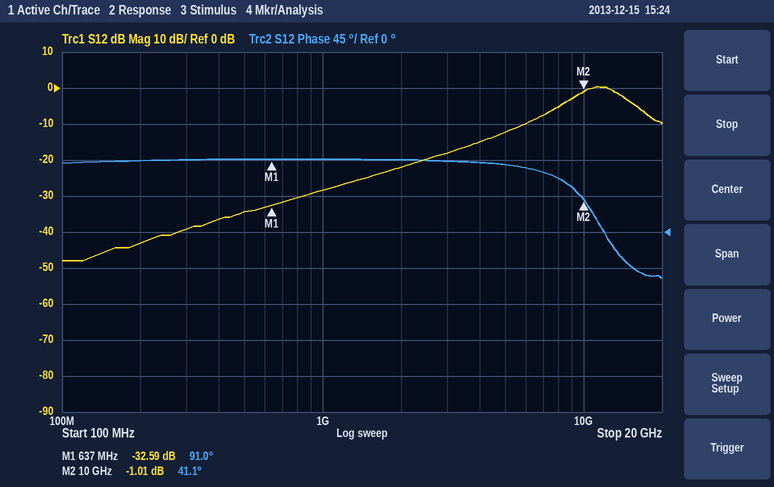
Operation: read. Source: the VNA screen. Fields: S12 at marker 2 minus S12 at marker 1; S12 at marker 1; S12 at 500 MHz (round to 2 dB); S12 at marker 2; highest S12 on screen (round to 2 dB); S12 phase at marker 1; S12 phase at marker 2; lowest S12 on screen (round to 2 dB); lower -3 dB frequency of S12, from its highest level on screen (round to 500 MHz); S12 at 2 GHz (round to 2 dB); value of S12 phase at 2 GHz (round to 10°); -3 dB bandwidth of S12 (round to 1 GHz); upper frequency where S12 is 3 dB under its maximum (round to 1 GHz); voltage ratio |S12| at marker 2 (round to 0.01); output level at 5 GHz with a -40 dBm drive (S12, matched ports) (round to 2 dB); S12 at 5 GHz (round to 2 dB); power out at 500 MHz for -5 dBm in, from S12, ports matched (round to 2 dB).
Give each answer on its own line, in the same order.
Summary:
31.58 dB
-32.59 dB
-34 dB
-1.01 dB
0 dB
91.0°
41.1°
-48 dB
9.0 GHz
-22 dB
90°
5 GHz
14 GHz
0.89
-52 dBm
-12 dB
-40 dBm
